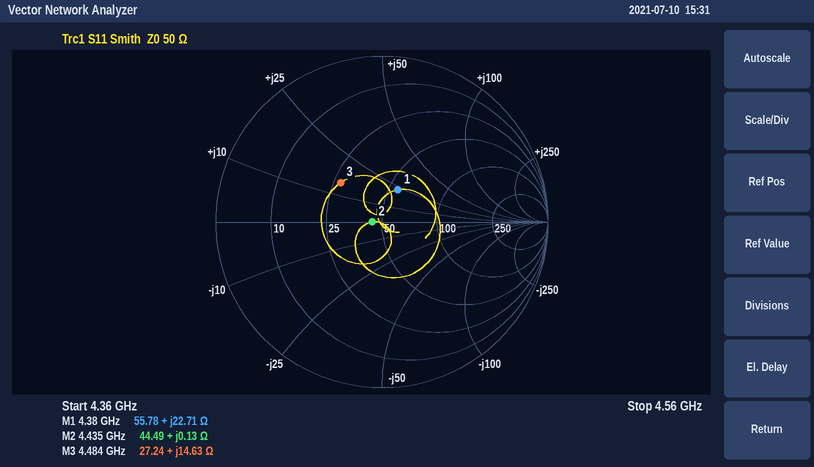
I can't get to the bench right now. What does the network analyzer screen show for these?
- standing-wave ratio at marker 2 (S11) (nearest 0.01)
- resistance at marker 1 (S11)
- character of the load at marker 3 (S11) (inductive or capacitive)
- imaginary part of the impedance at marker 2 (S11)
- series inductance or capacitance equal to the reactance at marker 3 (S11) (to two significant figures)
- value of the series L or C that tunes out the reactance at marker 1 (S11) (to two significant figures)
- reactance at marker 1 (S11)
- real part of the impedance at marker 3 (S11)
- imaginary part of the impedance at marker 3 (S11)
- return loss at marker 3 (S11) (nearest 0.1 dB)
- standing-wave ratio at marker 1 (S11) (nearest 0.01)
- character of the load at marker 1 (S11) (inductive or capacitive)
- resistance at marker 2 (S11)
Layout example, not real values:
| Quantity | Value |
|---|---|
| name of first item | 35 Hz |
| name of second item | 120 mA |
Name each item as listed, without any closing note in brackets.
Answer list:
| Quantity | Value |
|---|---|
| standing-wave ratio at marker 2 (S11) | 1.12 |
| resistance at marker 1 | 55.78 Ω |
| character of the load at marker 3 (S11) | inductive |
| imaginary part of the impedance at marker 2 | +0.13 Ω |
| series inductance or capacitance equal to the reactance at marker 3 (S11) | 520 pH |
| value of the series L or C that tunes out the reactance at marker 1 (S11) | 1.6 pF |
| reactance at marker 1 | +22.71 Ω |
| real part of the impedance at marker 3 | 27.24 Ω |
| imaginary part of the impedance at marker 3 | +14.63 Ω |
| return loss at marker 3 (S11) | 9.3 dB |
| standing-wave ratio at marker 1 (S11) | 1.55 |
| character of the load at marker 1 (S11) | inductive |
| resistance at marker 2 | 44.49 Ω |
